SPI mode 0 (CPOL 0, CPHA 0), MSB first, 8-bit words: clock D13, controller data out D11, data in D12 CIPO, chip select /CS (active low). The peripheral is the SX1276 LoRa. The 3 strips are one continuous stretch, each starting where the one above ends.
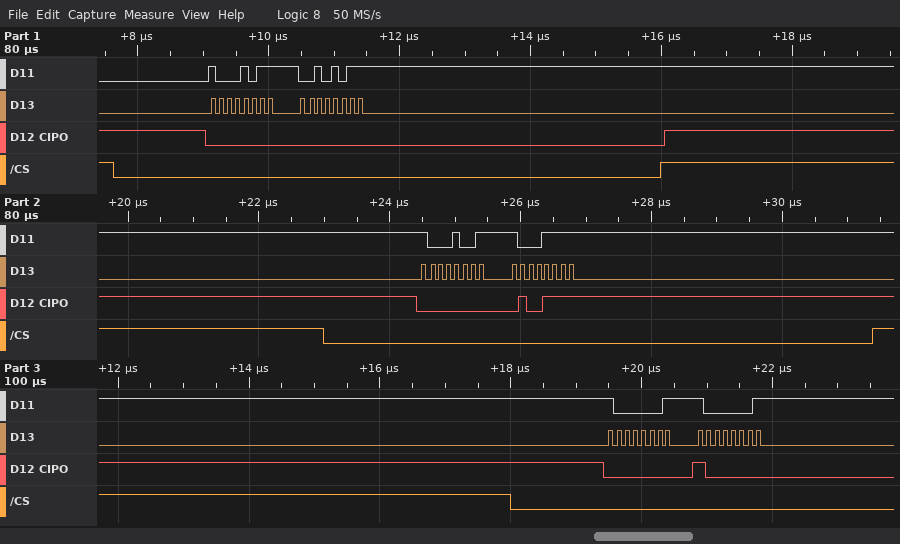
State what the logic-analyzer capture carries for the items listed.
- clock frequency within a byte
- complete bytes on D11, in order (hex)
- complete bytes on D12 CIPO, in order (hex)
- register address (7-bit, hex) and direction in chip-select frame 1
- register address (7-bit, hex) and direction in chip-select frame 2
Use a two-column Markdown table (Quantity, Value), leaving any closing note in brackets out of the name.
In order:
| Quantity | Value |
|---|---|
| clock frequency within a byte | 8 MHz |
| complete bytes on D11, in order | 8B 2B 89 8F 81 81 |
| complete bytes on D12 CIPO, in order | 00 00 00 4F 00 80 |
| register address (7-bit, hex) and direction in chip-select frame 1 | 0x0B write |
| register address (7-bit, hex) and direction in chip-select frame 2 | 0x09 write |
